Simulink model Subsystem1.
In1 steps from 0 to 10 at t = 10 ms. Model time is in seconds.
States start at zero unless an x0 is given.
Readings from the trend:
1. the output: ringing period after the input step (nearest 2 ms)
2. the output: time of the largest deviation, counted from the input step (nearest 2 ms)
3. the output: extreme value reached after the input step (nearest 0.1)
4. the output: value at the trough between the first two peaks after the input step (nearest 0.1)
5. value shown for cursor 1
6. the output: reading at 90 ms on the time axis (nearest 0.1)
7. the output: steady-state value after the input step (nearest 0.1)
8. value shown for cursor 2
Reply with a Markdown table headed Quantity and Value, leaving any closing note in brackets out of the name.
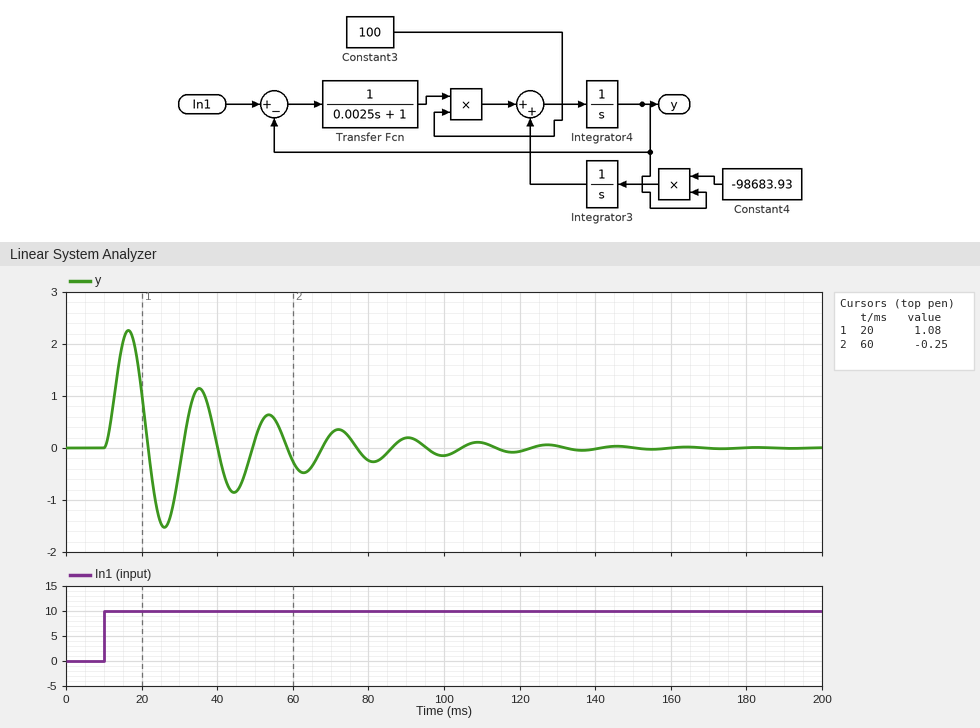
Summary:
| Quantity | Value |
|---|---|
| the output: ringing period after the input step | 18 ms |
| the output: time of the largest deviation, counted from the input step | 6 ms |
| the output: extreme value reached after the input step | 2.3 |
| the output: value at the trough between the first two peaks after the input step | -1.5 |
| value shown for cursor 1 | 1.08 |
| the output: reading at 90 ms on the time axis | 0.2 |
| the output: steady-state value after the input step | 0.0 |
| value shown for cursor 2 | -0.25 |
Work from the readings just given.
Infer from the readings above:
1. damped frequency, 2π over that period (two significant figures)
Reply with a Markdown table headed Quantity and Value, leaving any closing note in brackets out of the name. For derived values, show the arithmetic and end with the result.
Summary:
| Quantity | Value |
|---|---|
| damped frequency, 2π over that period | 2π / 18 = 0.35 rad/ms |
